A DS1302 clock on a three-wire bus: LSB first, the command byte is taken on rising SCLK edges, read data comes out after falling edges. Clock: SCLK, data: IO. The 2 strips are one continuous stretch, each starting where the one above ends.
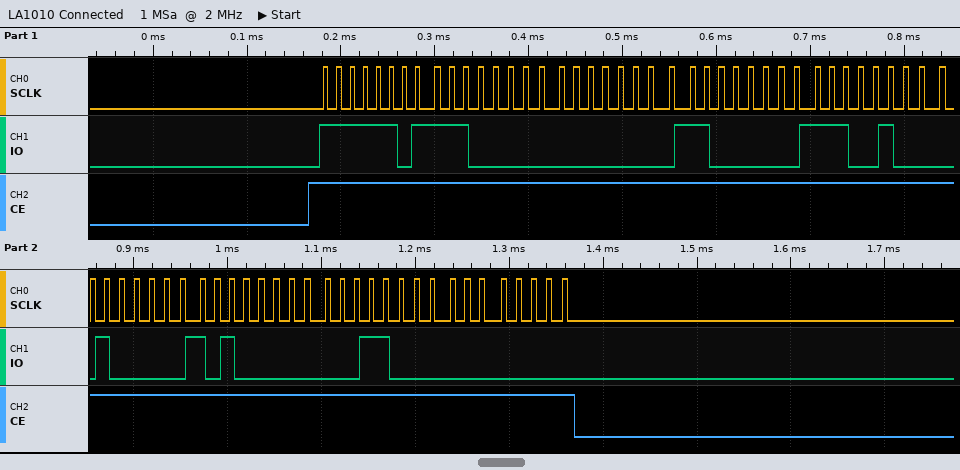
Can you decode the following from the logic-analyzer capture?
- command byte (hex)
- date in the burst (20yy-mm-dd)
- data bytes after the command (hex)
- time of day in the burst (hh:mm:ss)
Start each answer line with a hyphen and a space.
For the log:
- 0xBF
- 2018-04-27
- 07 00 03 27 04 05 18 00
- 03:00:07
